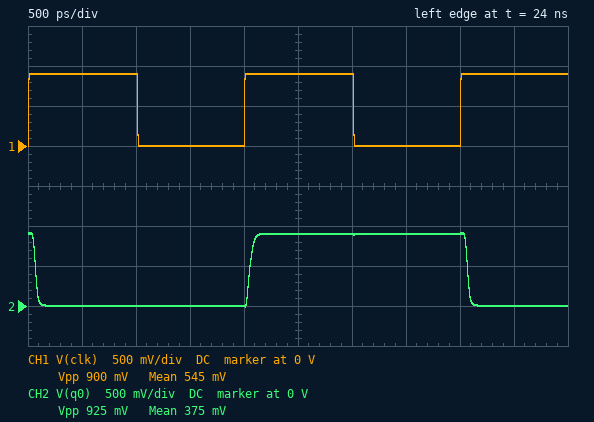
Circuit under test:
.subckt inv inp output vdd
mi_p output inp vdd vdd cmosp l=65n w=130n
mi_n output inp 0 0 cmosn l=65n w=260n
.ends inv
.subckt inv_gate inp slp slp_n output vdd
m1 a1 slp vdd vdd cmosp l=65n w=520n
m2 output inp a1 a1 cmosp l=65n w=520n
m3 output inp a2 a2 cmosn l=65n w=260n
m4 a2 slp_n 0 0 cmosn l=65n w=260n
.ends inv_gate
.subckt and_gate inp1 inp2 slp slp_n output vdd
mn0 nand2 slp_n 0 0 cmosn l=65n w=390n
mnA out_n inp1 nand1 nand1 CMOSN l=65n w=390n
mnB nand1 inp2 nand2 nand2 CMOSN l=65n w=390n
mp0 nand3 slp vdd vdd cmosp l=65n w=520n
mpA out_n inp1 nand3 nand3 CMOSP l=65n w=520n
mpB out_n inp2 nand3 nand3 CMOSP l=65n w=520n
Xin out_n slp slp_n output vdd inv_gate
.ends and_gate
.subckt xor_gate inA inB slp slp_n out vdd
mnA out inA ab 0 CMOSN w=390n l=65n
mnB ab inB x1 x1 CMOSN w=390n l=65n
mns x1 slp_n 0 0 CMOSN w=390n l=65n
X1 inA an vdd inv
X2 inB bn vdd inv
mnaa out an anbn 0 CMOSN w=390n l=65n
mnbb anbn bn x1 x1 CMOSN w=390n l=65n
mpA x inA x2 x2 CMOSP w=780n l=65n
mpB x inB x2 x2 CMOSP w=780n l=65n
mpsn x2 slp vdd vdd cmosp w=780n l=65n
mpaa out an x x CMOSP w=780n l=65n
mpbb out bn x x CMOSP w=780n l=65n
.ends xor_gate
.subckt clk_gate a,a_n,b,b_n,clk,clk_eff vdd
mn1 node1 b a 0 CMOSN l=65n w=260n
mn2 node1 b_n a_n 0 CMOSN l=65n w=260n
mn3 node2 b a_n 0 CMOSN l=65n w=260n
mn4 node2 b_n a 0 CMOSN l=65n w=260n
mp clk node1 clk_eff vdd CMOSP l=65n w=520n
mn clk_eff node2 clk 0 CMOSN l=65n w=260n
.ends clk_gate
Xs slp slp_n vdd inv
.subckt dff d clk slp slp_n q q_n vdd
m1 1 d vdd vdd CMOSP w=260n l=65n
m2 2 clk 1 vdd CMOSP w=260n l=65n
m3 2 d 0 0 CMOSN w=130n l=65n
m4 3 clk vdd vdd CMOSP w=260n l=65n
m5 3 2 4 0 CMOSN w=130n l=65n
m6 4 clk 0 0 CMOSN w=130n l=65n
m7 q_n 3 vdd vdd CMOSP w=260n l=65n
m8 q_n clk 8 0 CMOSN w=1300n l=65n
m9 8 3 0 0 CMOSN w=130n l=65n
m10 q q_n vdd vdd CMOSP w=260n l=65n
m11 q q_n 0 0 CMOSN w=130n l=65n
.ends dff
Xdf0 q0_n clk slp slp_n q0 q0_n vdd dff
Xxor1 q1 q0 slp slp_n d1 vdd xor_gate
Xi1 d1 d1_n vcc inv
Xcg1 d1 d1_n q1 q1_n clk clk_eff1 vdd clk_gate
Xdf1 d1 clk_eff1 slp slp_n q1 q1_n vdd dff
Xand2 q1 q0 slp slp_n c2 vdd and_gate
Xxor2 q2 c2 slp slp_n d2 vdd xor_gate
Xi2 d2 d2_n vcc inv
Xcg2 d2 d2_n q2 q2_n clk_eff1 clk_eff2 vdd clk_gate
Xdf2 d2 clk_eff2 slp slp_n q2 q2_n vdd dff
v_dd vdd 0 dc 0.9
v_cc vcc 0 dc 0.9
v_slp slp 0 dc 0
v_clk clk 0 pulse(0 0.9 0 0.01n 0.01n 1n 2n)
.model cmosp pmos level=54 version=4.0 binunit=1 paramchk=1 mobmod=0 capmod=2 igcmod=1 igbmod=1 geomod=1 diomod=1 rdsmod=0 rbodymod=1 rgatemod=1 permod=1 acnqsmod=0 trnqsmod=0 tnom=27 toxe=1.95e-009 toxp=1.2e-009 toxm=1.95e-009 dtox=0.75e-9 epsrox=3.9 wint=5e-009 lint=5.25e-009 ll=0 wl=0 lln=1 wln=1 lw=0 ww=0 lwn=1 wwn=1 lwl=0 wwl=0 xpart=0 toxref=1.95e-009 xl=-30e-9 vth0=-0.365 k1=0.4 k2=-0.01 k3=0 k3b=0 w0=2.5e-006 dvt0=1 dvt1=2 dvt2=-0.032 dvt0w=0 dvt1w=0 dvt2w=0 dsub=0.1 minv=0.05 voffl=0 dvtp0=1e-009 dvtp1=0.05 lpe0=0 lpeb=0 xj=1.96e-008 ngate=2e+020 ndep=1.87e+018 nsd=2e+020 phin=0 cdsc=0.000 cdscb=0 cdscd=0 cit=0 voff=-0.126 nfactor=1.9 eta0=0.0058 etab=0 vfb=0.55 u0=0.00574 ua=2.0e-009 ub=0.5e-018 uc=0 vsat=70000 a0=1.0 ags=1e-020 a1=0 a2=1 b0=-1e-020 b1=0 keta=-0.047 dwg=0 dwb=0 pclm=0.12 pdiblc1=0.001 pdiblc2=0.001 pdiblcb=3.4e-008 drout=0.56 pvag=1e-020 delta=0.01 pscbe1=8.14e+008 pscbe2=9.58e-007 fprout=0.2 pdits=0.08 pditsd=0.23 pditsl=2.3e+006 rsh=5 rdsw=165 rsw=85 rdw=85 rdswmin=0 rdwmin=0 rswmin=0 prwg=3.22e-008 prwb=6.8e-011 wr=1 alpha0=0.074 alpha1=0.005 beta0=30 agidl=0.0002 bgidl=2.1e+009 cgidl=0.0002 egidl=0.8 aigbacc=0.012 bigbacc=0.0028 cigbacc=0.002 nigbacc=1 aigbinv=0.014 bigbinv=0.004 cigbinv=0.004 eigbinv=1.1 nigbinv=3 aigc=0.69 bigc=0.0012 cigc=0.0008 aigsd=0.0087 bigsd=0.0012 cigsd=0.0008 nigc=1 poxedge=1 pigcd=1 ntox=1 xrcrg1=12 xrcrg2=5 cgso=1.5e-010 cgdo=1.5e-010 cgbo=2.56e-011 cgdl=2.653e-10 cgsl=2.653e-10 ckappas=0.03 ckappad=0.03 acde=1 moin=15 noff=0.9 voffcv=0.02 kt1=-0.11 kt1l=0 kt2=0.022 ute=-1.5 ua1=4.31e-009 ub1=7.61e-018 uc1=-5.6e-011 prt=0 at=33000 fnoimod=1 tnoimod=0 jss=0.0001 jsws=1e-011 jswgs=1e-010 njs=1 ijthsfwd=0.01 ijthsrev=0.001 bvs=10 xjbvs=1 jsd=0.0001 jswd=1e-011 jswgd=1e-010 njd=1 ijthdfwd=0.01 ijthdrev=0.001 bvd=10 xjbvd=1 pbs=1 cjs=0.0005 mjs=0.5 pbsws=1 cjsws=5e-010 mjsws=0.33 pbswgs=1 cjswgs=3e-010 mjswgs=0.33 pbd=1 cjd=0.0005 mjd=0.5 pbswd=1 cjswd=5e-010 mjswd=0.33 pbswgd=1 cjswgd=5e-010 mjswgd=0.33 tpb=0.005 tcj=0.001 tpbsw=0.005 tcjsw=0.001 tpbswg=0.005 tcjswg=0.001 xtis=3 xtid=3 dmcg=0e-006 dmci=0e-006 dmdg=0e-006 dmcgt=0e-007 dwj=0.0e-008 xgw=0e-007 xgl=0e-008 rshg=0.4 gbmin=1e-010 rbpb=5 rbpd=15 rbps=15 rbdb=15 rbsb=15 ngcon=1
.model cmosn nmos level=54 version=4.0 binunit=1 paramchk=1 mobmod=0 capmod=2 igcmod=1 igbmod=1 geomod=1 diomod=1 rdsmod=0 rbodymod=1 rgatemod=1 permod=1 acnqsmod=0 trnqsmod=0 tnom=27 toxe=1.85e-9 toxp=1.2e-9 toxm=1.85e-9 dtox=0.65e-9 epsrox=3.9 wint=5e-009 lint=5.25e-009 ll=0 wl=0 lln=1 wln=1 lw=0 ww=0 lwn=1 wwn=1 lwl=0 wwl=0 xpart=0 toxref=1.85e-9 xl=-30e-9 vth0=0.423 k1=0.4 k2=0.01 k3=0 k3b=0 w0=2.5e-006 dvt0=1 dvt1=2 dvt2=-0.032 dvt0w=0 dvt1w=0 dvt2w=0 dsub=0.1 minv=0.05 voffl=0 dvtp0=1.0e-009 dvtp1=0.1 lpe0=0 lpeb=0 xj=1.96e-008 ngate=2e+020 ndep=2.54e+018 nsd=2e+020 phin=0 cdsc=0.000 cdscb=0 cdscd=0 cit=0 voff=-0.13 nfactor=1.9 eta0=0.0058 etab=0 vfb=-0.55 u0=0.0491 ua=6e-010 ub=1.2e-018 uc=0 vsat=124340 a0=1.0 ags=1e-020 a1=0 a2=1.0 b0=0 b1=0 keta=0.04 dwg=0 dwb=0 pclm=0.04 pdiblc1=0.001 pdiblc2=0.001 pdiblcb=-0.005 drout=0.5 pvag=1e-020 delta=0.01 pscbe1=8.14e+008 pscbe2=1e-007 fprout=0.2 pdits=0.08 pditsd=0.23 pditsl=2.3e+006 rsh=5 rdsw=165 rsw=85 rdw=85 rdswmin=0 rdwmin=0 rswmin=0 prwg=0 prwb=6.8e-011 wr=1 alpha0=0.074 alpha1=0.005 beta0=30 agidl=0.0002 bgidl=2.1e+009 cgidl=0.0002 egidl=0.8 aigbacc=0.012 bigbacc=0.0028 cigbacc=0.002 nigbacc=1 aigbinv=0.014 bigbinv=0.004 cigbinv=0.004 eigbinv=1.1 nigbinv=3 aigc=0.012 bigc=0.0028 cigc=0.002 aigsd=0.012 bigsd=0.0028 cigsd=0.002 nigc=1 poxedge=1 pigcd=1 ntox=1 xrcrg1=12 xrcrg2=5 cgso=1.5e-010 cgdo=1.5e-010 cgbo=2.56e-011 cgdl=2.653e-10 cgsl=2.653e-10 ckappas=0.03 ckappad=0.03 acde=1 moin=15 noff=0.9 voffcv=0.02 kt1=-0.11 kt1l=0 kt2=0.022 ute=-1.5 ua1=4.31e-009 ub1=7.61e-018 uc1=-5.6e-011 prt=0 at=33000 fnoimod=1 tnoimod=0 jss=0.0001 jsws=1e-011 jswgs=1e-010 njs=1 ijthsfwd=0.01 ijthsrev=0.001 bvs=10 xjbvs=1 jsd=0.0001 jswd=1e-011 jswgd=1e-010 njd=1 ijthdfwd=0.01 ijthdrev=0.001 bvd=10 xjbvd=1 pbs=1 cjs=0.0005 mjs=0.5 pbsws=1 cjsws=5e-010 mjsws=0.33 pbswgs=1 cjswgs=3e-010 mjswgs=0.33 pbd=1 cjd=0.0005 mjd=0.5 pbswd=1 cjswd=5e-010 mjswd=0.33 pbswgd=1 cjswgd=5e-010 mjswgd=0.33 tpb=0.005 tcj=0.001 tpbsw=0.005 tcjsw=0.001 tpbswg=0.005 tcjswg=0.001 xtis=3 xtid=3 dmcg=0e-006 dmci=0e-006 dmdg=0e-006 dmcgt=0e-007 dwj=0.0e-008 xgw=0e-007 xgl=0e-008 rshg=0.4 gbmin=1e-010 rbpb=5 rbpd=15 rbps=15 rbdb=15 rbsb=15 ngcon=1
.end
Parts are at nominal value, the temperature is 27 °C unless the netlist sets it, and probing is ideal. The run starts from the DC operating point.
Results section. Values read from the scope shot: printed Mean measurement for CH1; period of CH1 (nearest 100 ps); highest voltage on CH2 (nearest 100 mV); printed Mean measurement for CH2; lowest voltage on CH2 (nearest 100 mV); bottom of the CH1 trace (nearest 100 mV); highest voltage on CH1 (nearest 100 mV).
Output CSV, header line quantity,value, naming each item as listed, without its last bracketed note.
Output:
quantity,value
printed Mean measurement for CH1,545 mV
period of CH1,2.0 ns
highest voltage on CH2,900 mV
printed Mean measurement for CH2,375 mV
lowest voltage on CH2,0 V
bottom of the CH1 trace,0 V
highest voltage on CH1,900 mV
